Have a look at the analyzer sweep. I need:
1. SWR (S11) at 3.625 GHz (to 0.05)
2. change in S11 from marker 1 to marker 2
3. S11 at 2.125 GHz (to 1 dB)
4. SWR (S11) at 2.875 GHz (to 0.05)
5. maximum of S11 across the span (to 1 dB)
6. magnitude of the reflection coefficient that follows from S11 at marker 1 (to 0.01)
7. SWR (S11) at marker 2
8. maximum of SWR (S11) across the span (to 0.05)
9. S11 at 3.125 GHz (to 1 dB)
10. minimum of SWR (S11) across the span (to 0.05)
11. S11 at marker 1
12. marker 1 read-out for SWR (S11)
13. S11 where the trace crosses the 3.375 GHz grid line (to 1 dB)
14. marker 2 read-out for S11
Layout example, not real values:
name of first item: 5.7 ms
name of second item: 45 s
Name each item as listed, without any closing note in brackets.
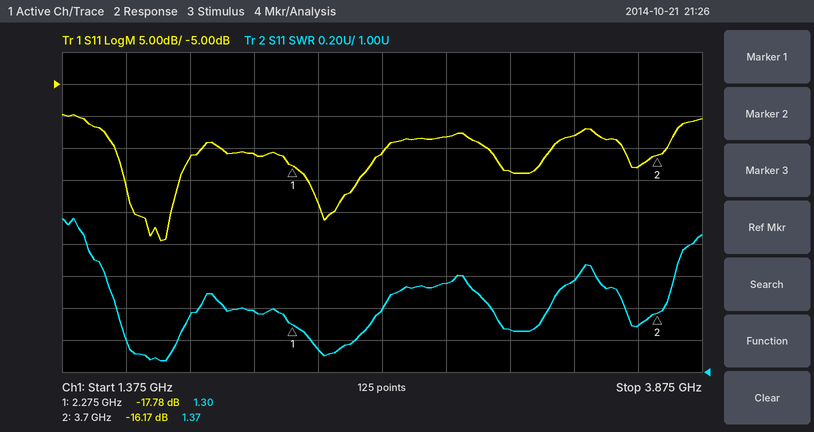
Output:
SWR (S11) at 3.625 GHz: 1.30
change in S11 from marker 1 to marker 2: 1.61 dB
S11 at 2.125 GHz: -16 dB
SWR (S11) at 2.875 GHz: 1.55
maximum of S11 across the span: -10 dB
magnitude of the reflection coefficient that follows from S11 at marker 1: 0.13
SWR (S11) at marker 2: 1.37
maximum of SWR (S11) across the span: 1.95
S11 at 3.125 GHz: -19 dB
minimum of SWR (S11) across the span: 1.05
S11 at marker 1: -17.78 dB
marker 1 read-out for SWR: 1.30
S11 where the trace crosses the 3.375 GHz grid line: -13 dB
marker 2 read-out for S11: -16.17 dB
